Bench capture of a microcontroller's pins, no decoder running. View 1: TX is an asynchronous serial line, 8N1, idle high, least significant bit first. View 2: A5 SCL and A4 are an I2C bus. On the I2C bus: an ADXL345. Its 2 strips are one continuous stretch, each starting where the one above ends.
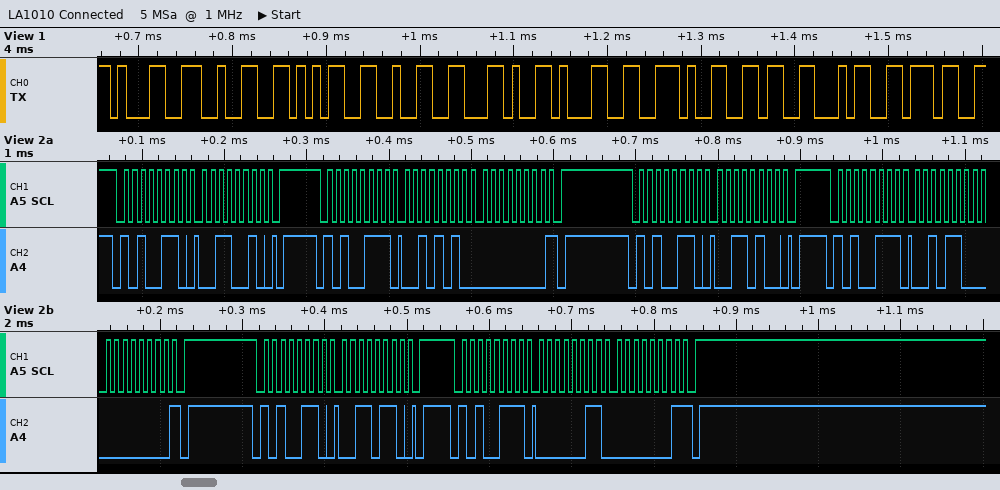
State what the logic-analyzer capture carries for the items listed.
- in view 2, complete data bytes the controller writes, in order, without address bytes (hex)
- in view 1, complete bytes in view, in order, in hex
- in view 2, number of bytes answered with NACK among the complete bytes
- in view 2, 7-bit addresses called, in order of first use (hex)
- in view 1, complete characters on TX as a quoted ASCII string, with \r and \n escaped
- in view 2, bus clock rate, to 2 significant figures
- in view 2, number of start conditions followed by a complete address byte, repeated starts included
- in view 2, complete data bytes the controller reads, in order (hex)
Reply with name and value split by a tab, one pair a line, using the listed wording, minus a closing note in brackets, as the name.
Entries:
in view 2, complete data bytes the controller writes, in order, without address bytes	32 34 36
in view 1, complete bytes in view, in order, in hex	31 32 35 32 2C 31 2E 36 34 37
in view 2, number of bytes answered with NACK among the complete bytes	3
in view 2, 7-bit addresses called, in order of first use	0x53
in view 1, complete characters on TX as a quoted ASCII string, with \r and \n escaped	"1252,1.647"
in view 2, bus clock rate, to 2 significant figures	100 kHz
in view 2, number of start conditions followed by a complete address byte, repeated starts included	6
in view 2, complete data bytes the controller reads, in order	2A 00 2C 00 03 01
